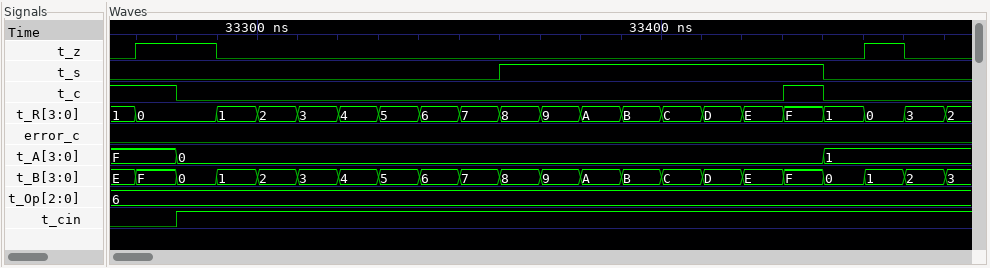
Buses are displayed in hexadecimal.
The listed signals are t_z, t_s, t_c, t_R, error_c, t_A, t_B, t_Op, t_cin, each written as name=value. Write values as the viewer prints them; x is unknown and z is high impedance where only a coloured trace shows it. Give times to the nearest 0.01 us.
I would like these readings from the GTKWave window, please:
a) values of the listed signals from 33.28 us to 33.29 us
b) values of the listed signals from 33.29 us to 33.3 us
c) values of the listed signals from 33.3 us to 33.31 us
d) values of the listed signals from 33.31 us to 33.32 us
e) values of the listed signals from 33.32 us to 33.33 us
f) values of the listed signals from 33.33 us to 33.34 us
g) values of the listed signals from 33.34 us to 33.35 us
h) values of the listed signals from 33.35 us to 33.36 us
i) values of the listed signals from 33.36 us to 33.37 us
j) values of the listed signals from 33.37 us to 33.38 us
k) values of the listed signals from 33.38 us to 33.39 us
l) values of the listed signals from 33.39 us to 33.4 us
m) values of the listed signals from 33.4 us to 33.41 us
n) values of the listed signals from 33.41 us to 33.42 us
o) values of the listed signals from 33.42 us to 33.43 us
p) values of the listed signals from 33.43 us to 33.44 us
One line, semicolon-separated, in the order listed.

t_z=1, t_s=0, t_c=0, t_R=0, error_c=0, t_A=0, t_B=0, t_Op=6, t_cin=1; t_z=0, t_s=0, t_c=0, t_R=1, error_c=0, t_A=0, t_B=1, t_Op=6, t_cin=1; t_z=0, t_s=0, t_c=0, t_R=2, error_c=0, t_A=0, t_B=2, t_Op=6, t_cin=1; t_z=0, t_s=0, t_c=0, t_R=3, error_c=0, t_A=0, t_B=3, t_Op=6, t_cin=1; t_z=0, t_s=0, t_c=0, t_R=4, error_c=0, t_A=0, t_B=4, t_Op=6, t_cin=1; t_z=0, t_s=0, t_c=0, t_R=5, error_c=0, t_A=0, t_B=5, t_Op=6, t_cin=1; t_z=0, t_s=0, t_c=0, t_R=6, error_c=0, t_A=0, t_B=6, t_Op=6, t_cin=1; t_z=0, t_s=0, t_c=0, t_R=7, error_c=0, t_A=0, t_B=7, t_Op=6, t_cin=1; t_z=0, t_s=1, t_c=0, t_R=8, error_c=0, t_A=0, t_B=8, t_Op=6, t_cin=1; t_z=0, t_s=1, t_c=0, t_R=9, error_c=0, t_A=0, t_B=9, t_Op=6, t_cin=1; t_z=0, t_s=1, t_c=0, t_R=A, error_c=0, t_A=0, t_B=A, t_Op=6, t_cin=1; t_z=0, t_s=1, t_c=0, t_R=B, error_c=0, t_A=0, t_B=B, t_Op=6, t_cin=1; t_z=0, t_s=1, t_c=0, t_R=C, error_c=0, t_A=0, t_B=C, t_Op=6, t_cin=1; t_z=0, t_s=1, t_c=0, t_R=D, error_c=0, t_A=0, t_B=D, t_Op=6, t_cin=1; t_z=0, t_s=1, t_c=0, t_R=E, error_c=0, t_A=0, t_B=E, t_Op=6, t_cin=1; t_z=0, t_s=1, t_c=1, t_R=F, error_c=0, t_A=0, t_B=F, t_Op=6, t_cin=1
